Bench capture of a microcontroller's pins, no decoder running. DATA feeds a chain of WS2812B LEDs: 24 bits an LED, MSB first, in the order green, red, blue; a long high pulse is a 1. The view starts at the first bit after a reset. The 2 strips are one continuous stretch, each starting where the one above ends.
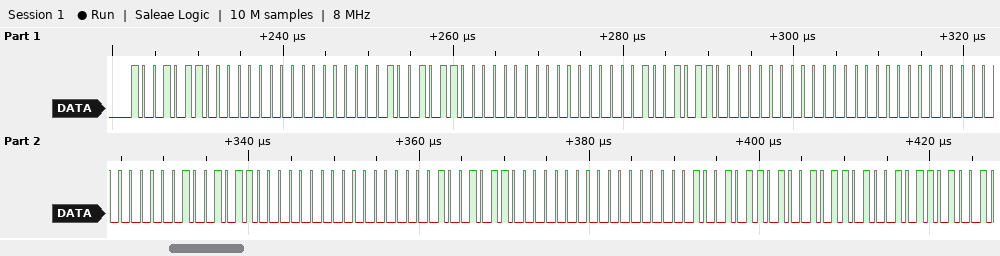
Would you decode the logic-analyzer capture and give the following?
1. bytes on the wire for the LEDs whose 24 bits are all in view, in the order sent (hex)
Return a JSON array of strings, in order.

["96 00 00 96 00 00 96 00 00 00 00 96 00 00 96 00 00 96"]
